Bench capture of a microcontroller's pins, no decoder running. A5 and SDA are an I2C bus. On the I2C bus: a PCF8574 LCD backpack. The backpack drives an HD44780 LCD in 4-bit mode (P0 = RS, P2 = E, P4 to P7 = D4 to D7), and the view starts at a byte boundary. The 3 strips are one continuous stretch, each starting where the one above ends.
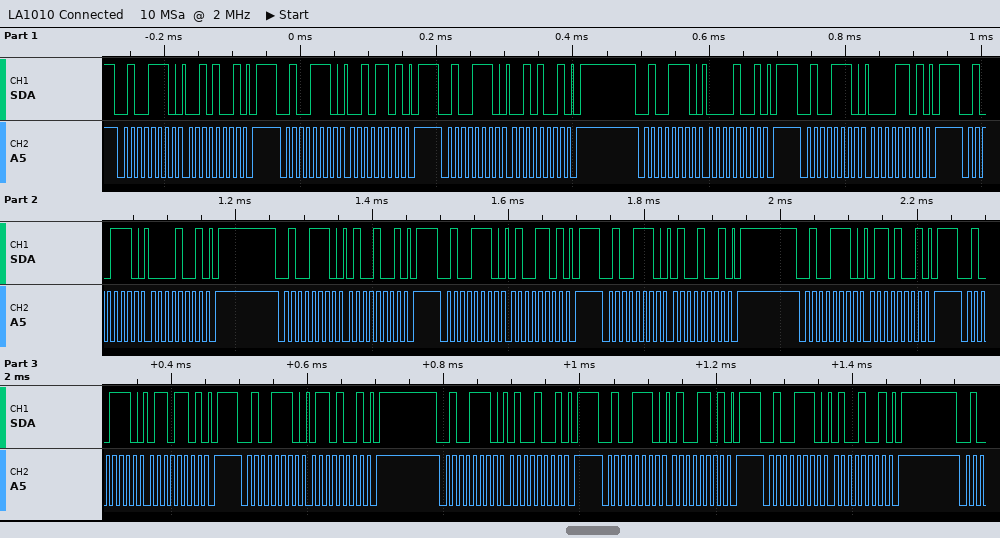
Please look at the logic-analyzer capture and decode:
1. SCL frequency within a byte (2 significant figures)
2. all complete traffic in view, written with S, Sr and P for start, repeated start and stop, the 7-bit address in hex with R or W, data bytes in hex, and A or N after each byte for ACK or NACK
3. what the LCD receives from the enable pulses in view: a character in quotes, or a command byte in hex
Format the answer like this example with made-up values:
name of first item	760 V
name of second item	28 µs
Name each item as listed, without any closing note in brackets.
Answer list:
SCL frequency within a byte	100 kHz
all complete traffic in view, written with S, Sr and P for start, repeated start and stop, the 7-bit address in hex with R or W, data bytes in hex, and A or N after each byte for ACK or NACK	S 27W A 29 A P S 27W A 2D A P S 27W A 29 A P S 27W A 09 A P S 27W A 0D A P S 27W A 09 A P S 27W A 49 A P S 27W A 4D A P S 27W A 49 A P S 27W A 69 A P S 27W A 6D A P S 27W A 69 A P S 27W A 49 A P S 27W A 4D A P S 27W A 49 A P
what the LCD receives from the enable pulses in view: a character in quotes, or a command byte in hex	' ' 'F'
